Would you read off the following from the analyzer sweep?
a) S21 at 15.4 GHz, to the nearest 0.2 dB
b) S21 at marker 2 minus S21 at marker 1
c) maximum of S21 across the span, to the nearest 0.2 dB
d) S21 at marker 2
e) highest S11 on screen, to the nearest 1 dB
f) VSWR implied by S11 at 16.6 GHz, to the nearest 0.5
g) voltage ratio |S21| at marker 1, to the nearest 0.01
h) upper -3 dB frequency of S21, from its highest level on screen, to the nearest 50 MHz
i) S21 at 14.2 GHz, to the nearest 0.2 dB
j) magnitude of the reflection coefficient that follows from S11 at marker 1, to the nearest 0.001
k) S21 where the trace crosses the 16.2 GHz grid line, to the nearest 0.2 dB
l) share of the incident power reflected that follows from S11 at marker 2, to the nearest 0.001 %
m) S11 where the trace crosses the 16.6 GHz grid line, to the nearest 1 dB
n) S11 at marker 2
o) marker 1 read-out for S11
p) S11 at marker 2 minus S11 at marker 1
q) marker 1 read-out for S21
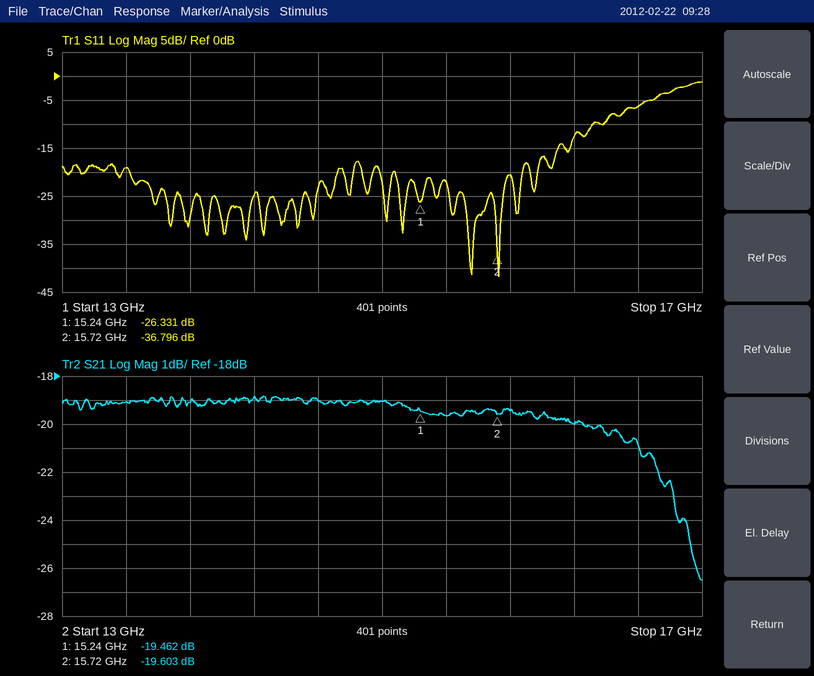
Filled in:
-19.6 dB
-0.141 dB
-18.8 dB
-19.603 dB
-1 dB
3.0
0.11
16.70 GHz
-18.8 dB
0.048
-20.0 dB
0.021 %
-6 dB
-36.796 dB
-26.331 dB
-10.465 dB
-19.462 dB
